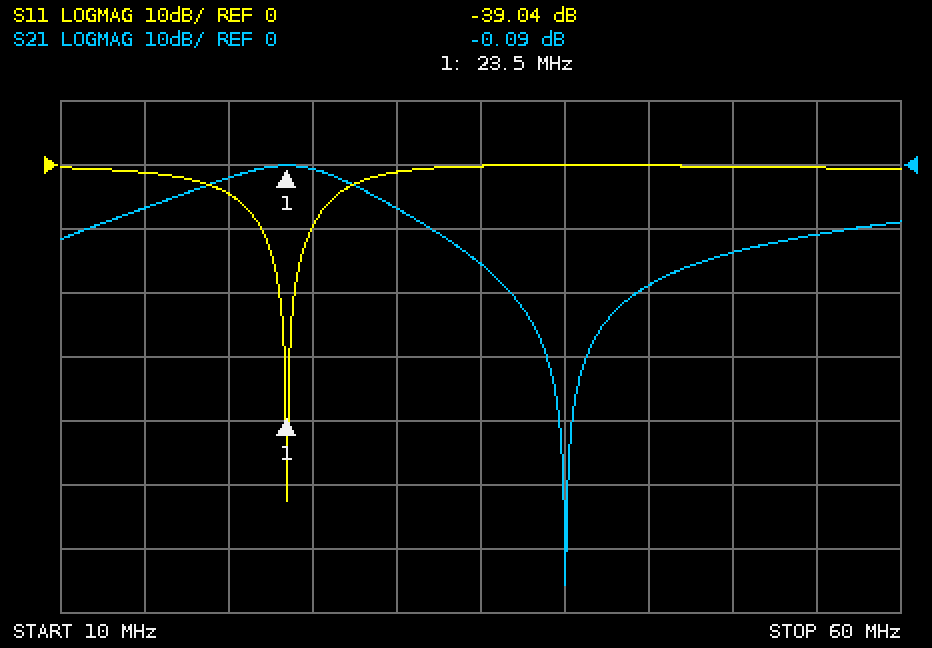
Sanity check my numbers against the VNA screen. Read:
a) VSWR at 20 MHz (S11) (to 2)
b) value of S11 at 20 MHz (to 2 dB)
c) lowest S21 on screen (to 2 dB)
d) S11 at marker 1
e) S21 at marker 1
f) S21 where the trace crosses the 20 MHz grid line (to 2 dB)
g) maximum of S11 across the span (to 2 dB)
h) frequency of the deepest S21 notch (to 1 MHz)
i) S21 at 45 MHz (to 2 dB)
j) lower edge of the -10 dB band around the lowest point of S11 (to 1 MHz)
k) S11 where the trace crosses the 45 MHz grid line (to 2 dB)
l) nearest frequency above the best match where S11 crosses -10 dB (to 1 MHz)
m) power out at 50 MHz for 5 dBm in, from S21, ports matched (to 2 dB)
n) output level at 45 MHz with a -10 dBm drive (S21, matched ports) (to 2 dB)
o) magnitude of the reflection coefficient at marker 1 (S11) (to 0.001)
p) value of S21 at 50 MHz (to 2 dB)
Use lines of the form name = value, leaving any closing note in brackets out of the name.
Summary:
VSWR at 20 MHz (S11) = 4
value of S11 at 20 MHz = -4 dB
lowest S21 on screen = -66 dB
S11 at marker 1 = -39.04 dB
S21 at marker 1 = -0.09 dB
S21 where the trace crosses the 20 MHz grid line = -2 dB
maximum of S11 across the span = 0 dB
frequency of the deepest S21 notch = 40 MHz
S21 at 45 MHz = -18 dB
lower edge of the -10 dB band around the lowest point of S11 = 22 MHz
S11 where the trace crosses the 45 MHz grid line = 0 dB
nearest frequency above the best match where S11 crosses -10 dB = 25 MHz
power out at 50 MHz for 5 dBm in, from S21, ports matched = -8 dBm
output level at 45 MHz with a -10 dBm drive (S21, matched ports) = -28 dBm
magnitude of the reflection coefficient at marker 1 (S11) = 0.011
value of S21 at 50 MHz = -14 dB
